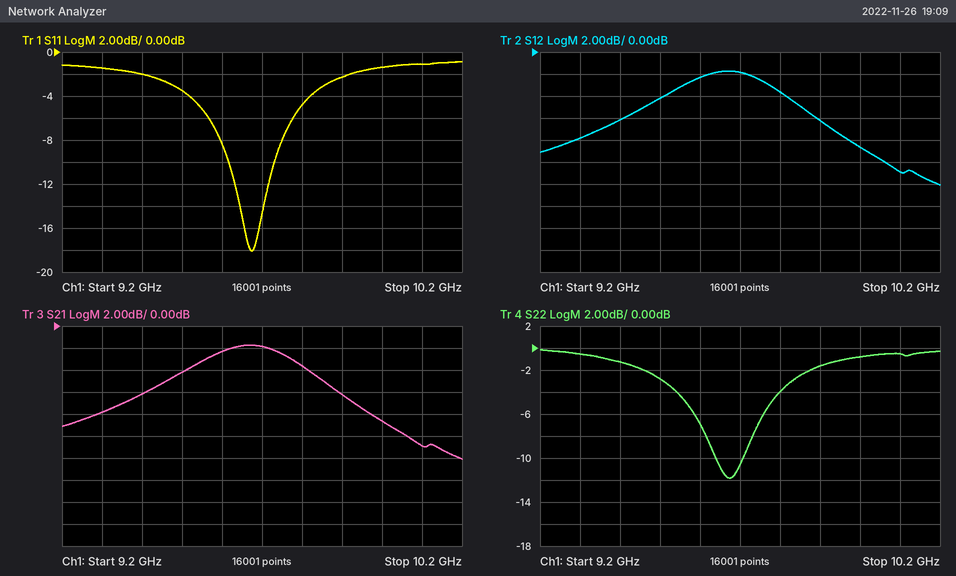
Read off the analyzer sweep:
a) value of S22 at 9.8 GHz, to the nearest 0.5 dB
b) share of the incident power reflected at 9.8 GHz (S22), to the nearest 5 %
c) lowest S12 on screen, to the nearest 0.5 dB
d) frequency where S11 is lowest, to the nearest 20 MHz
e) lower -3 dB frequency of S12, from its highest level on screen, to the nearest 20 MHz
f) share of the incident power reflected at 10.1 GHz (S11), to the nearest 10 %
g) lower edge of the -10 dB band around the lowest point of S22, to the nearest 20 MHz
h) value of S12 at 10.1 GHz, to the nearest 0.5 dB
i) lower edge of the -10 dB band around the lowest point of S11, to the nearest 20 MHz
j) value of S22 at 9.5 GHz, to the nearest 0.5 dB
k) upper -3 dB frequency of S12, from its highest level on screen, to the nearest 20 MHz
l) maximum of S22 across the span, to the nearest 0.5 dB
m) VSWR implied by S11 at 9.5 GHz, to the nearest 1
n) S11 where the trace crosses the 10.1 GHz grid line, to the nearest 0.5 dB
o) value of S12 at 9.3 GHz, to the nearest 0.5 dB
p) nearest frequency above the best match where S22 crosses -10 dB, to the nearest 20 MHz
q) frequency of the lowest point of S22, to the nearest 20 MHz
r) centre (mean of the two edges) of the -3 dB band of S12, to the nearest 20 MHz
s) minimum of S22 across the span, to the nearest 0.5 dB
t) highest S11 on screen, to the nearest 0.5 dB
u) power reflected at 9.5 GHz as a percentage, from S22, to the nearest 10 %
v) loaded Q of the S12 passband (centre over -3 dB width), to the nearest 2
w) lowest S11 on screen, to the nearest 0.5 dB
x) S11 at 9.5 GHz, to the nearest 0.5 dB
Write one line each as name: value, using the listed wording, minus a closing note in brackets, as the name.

value of S22 at 9.8 GHz, to the nearest 0.5 dB: -4.0 dB
share of the incident power reflected at 9.8 GHz (S22), to the nearest 5 %: 40 %
lowest S12 on screen, to the nearest 0.5 dB: -12.0 dB
frequency where S11 is lowest, to the nearest 20 MHz: 9.68 GHz
lower -3 dB frequency of S12, from its highest level on screen, to the nearest 20 MHz: 9.48 GHz
share of the incident power reflected at 10.1 GHz (S11), to the nearest 10 %: 80 %
lower edge of the -10 dB band around the lowest point of S22, to the nearest 20 MHz: 9.64 GHz
value of S12 at 10.1 GHz, to the nearest 0.5 dB: -11.0 dB
lower edge of the -10 dB band around the lowest point of S11, to the nearest 20 MHz: 9.62 GHz
value of S22 at 9.5 GHz, to the nearest 0.5 dB: -3.0 dB
upper -3 dB frequency of S12, from its highest level on screen, to the nearest 20 MHz: 9.84 GHz
maximum of S22 across the span, to the nearest 0.5 dB: 0.0 dB
VSWR implied by S11 at 9.5 GHz, to the nearest 1: 5
S11 where the trace crosses the 10.1 GHz grid line, to the nearest 0.5 dB: -1.0 dB
value of S12 at 9.3 GHz, to the nearest 0.5 dB: -8.0 dB
nearest frequency above the best match where S22 crosses -10 dB, to the nearest 20 MHz: 9.70 GHz
frequency of the lowest point of S22, to the nearest 20 MHz: 9.68 GHz
centre (mean of the two edges) of the -3 dB band of S12, to the nearest 20 MHz: 9.66 GHz
minimum of S22 across the span, to the nearest 0.5 dB: -12.0 dB
highest S11 on screen, to the nearest 0.5 dB: -1.0 dB
power reflected at 9.5 GHz as a percentage, from S22, to the nearest 10 %: 50 %
loaded Q of the S12 passband (centre over -3 dB width), to the nearest 2: 26
lowest S11 on screen, to the nearest 0.5 dB: -18.0 dB
S11 at 9.5 GHz, to the nearest 0.5 dB: -3.5 dB
